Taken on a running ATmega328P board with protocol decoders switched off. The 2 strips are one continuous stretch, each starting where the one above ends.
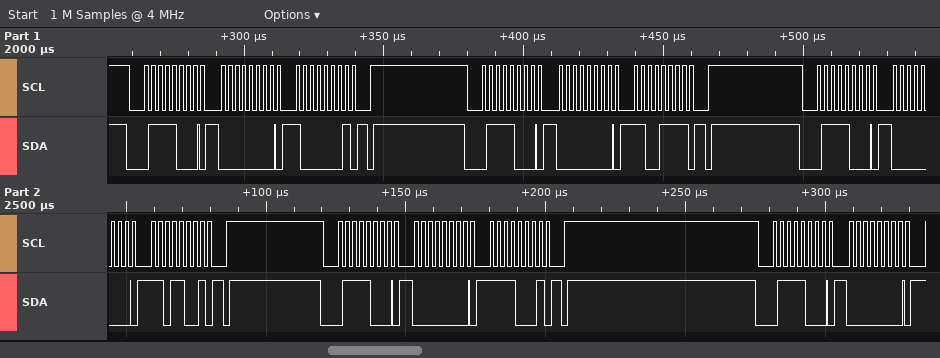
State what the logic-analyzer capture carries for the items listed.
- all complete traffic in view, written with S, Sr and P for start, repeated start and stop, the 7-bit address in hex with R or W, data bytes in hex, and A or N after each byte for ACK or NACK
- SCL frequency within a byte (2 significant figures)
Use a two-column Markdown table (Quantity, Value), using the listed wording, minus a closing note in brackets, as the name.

| Quantity | Value |
|---|---|
| all complete traffic in view, written with S, Sr and P for start, repeated start and stop, the 7-bit address in hex with R or W, data bytes in hex, and A or N after each byte for ACK or NACK | S 3CW A 00 A 81 A P S 3CW A 00 A CF A P S 3CW A 00 A D9 A P S 3CW A 00 A F1 A P S 3CW A 00 A |
| SCL frequency within a byte | 400 kHz |
